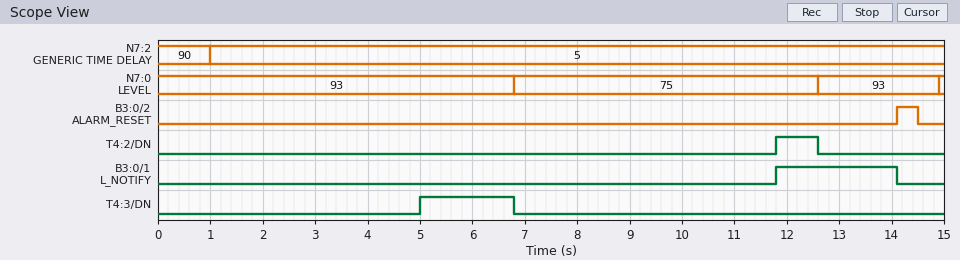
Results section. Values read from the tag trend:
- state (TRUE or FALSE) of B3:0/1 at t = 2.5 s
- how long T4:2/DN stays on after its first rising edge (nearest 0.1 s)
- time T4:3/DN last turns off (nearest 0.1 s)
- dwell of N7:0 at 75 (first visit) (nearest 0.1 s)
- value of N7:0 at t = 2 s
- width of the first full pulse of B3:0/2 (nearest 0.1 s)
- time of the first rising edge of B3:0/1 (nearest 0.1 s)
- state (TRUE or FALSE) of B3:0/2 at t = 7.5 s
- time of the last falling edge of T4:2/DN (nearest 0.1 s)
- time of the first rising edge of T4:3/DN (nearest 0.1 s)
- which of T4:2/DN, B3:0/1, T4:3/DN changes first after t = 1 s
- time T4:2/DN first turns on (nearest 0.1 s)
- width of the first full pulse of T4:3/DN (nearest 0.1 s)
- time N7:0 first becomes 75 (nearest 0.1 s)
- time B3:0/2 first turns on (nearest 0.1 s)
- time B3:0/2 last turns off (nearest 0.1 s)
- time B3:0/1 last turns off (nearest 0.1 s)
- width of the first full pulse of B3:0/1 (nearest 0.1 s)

FALSE
0.8 s
6.8 s
5.8 s
93
0.4 s
11.8 s
FALSE
12.6 s
5.0 s
T4:3/DN
11.8 s
1.8 s
6.8 s
14.1 s
14.5 s
14.1 s
2.3 s
